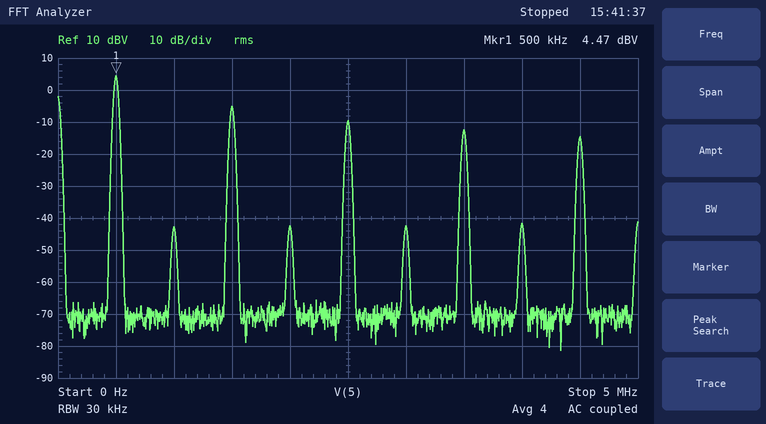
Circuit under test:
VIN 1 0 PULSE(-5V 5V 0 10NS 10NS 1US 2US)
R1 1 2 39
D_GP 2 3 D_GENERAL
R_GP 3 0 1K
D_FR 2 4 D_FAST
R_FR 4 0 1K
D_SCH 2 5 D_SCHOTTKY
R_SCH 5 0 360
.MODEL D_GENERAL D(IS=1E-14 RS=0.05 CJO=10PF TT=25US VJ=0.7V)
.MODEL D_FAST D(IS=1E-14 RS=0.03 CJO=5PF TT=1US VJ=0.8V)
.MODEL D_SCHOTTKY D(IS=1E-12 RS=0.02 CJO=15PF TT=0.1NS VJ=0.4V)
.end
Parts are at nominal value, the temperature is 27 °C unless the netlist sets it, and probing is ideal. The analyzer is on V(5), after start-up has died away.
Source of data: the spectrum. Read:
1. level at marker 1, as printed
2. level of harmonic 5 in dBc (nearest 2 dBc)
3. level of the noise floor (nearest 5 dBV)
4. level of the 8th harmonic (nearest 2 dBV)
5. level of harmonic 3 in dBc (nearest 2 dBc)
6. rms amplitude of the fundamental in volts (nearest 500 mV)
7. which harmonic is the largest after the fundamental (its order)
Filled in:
4.47 dBV
-14 dBc
-70 dBV
-42 dBV
-10 dBc
1.5 V
3
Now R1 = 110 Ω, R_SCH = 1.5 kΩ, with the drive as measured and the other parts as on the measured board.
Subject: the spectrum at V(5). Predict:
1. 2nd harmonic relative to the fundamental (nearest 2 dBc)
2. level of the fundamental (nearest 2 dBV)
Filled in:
-42 dBc
4 dBV
